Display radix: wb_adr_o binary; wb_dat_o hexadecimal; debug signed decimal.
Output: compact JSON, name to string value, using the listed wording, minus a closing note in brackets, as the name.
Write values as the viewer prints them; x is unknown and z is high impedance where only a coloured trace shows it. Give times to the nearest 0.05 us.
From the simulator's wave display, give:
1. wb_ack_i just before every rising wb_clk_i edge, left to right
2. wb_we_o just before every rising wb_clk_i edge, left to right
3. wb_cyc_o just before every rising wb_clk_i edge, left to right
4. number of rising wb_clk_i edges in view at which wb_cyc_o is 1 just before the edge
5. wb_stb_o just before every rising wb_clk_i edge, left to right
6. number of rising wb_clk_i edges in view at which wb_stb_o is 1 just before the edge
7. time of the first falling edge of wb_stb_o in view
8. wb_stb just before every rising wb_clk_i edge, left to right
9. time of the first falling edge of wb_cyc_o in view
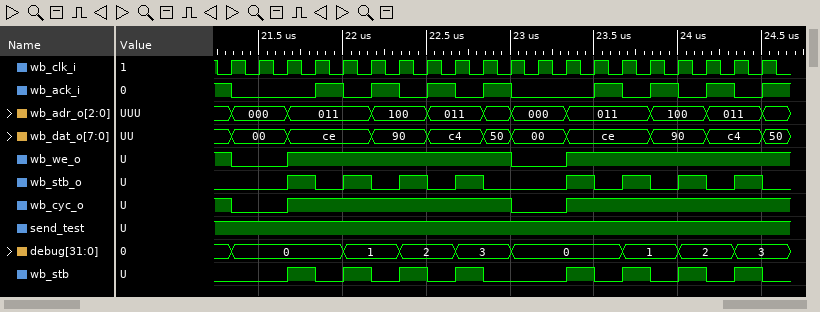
{"wb_ack_i just before every rising wb_clk_i edge, left to right": "1 0 0 0 1 0 1 0 1 0 1 0 0 0 1 0 1 0 1 0", "wb_we_o just before every rising wb_clk_i edge, left to right": "1 0 0 1 1 1 1 1 1 1 1 0 0 1 1 1 1 1 1 1", "wb_cyc_o just before every rising wb_clk_i edge, left to right": "1 0 0 1 1 1 1 1 1 1 1 0 0 1 1 1 1 1 1 1", "number of rising wb_clk_i edges in view at which wb_cyc_o is 1 just before the edge": "16", "wb_stb_o just before every rising wb_clk_i edge, left to right": "0 0 0 1 0 1 0 1 0 1 0 0 0 1 0 1 0 1 0 1", "number of rising wb_clk_i edges in view at which wb_stb_o is 1 just before the edge": "8", "time of the first falling edge of wb_stb_o in view": "21.85 us", "wb_stb just before every rising wb_clk_i edge, left to right": "0 0 0 1 0 1 0 1 0 1 0 0 0 1 0 1 0 1 0 1", "time of the first falling edge of wb_cyc_o in view": "21.35 us"}
